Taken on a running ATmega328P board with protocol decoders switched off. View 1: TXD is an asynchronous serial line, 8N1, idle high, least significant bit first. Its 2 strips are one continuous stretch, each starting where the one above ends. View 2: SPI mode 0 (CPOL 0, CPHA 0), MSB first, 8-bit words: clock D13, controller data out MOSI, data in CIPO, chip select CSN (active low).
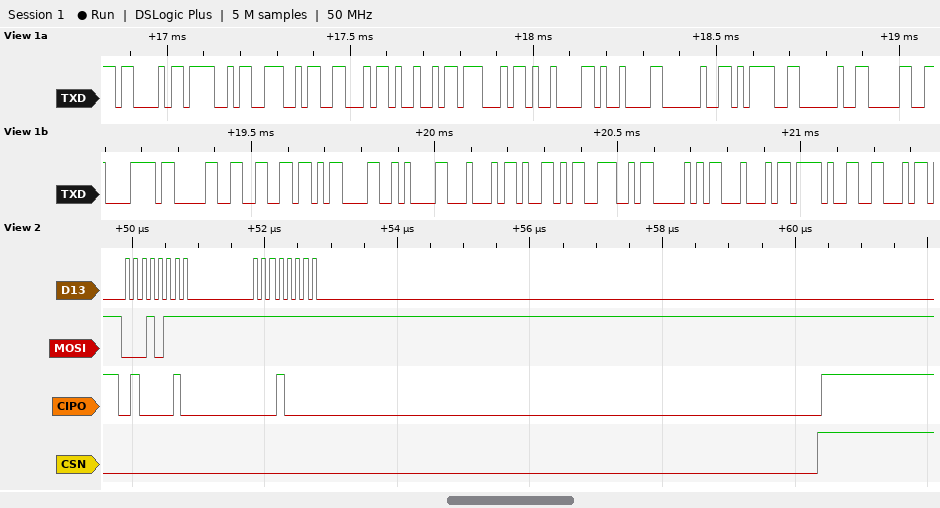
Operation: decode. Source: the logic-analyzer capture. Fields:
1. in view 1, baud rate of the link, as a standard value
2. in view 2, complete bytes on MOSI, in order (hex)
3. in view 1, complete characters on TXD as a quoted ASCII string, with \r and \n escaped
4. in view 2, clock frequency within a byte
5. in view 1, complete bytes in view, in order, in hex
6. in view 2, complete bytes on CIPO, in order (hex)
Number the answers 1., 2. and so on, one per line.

1. 57600 baud
2. 0x17 0xFF
3. "CONFIG\t\t = 0x0f\r\nDYNPD/F"
4. 8 MHz
5. 0x43 0x4F 0x4E 0x46 0x49 0x47 0x09 0x09 0x20 0x3D 0x20 0x30 0x78 0x30 0x66 0x0D 0x0A 0x44 0x59 0x4E 0x50 0x44 0x2F 0x46
6. 0x42 0x10
